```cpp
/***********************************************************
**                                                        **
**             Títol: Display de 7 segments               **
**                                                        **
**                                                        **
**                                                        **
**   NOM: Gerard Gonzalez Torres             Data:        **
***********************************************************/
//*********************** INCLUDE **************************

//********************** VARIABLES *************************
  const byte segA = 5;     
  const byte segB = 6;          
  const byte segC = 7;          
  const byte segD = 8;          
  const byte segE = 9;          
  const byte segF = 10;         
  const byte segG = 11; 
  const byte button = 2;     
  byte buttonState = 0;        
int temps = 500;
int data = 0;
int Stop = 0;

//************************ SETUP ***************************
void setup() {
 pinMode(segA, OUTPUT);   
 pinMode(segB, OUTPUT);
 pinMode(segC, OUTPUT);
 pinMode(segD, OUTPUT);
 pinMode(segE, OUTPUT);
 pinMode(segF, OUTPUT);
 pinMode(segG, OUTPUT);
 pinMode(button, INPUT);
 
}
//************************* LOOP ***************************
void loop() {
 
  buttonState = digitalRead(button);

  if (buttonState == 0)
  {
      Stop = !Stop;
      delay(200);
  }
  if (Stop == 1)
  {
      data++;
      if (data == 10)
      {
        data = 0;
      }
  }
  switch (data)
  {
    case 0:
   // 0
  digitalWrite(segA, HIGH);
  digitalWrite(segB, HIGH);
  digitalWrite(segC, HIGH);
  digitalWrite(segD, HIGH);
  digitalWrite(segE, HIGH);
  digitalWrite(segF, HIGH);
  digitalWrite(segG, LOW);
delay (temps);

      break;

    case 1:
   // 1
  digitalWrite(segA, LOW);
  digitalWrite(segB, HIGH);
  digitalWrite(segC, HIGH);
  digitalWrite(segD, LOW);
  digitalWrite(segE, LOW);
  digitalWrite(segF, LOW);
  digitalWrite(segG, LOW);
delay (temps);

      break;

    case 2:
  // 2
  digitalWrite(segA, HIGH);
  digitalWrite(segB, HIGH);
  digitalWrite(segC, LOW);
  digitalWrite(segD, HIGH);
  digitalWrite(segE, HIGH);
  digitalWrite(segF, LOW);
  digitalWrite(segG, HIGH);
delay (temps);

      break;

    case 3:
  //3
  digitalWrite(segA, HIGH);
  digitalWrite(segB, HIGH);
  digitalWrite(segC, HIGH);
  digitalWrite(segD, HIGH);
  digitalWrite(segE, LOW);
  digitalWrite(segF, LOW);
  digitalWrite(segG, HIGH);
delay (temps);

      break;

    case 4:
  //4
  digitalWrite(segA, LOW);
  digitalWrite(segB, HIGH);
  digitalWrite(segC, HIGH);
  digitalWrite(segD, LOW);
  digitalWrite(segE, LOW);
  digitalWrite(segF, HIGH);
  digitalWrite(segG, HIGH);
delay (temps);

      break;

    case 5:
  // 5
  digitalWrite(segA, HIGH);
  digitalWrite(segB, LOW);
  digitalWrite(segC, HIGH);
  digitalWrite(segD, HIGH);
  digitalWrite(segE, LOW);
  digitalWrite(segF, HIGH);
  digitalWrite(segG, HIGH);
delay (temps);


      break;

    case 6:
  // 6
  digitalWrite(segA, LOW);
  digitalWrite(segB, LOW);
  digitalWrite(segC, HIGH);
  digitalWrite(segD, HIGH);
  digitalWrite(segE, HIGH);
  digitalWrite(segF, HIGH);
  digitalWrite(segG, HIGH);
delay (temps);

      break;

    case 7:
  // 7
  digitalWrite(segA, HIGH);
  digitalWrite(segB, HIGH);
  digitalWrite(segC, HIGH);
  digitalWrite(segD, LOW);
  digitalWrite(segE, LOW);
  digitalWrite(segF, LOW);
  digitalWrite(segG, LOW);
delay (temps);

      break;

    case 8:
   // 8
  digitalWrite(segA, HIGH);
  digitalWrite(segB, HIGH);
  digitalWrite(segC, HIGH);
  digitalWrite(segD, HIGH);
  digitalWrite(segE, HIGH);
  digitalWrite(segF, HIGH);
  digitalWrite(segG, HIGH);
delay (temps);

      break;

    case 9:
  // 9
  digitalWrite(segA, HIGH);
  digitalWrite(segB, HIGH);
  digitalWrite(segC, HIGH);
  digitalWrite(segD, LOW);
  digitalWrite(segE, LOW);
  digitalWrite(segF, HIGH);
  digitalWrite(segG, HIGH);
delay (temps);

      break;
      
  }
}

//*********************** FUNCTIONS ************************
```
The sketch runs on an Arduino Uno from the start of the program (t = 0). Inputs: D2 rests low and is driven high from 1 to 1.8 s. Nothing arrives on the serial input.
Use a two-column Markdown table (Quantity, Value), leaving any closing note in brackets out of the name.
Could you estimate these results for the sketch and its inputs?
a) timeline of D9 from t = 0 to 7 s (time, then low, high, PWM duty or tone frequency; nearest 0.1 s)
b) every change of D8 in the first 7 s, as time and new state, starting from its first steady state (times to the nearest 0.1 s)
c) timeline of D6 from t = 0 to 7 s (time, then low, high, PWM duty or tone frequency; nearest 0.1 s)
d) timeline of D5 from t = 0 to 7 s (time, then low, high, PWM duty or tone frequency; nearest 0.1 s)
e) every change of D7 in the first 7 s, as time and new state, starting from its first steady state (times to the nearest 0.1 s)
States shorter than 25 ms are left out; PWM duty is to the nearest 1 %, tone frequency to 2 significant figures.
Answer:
| Quantity | Value |
|---|---|
| timeline of D9 from t = 0 to 7 s | 0 s low; 2.1 s high; 3.5 s low |
| every change of D8 in the first 7 s, as time and new state, starting from its first steady state | 0 s low; 2.1 s high; 4.9 s low; 6.3 s high |
| timeline of D6 from t = 0 to 7 s | 0 s low; 0.2 s high; 6.3 s low |
| timeline of D5 from t = 0 to 7 s | 0 s low; 2.1 s high; 4.9 s low; 6.3 s high |
| every change of D7 in the first 7 s, as time and new state, starting from its first steady state | 0 s low; 0.2 s high; 2.1 s low; 3.5 s high |
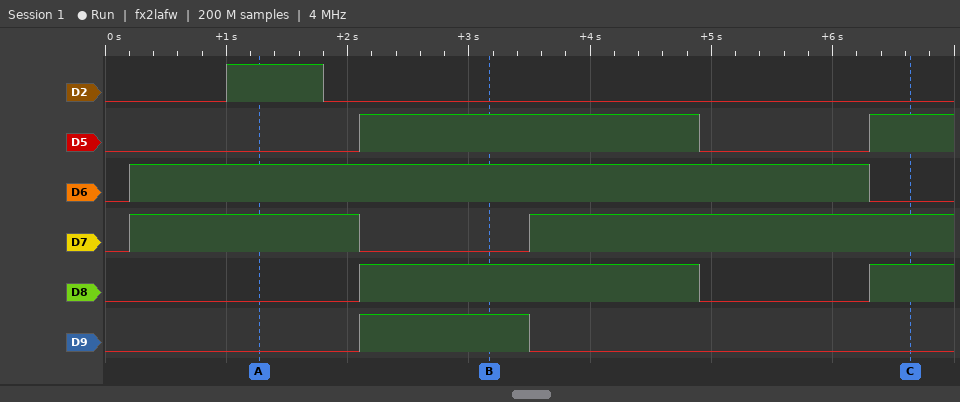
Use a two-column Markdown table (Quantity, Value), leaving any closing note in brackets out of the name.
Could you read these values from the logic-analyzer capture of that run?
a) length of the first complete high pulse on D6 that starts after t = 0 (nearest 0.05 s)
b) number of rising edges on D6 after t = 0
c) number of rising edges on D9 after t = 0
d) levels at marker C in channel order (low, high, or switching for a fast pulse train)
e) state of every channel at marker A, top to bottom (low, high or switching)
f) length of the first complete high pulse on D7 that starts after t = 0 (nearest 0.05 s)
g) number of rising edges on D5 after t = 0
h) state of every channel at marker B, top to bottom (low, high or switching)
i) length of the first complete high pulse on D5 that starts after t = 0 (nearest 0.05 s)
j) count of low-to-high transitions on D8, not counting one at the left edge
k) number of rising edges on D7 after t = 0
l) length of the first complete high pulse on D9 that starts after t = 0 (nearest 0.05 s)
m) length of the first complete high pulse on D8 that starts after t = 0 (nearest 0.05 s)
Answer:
| Quantity | Value |
|---|---|
| length of the first complete high pulse on D6 that starts after t = 0 | 6.10 s |
| number of rising edges on D6 after t = 0 | 1 |
| number of rising edges on D9 after t = 0 | 1 |
| levels at marker C in channel order | D2 low, D5 high, D6 low, D7 high, D8 high, D9 low |
| state of every channel at marker A, top to bottom | D2 high, D5 low, D6 high, D7 high, D8 low, D9 low |
| length of the first complete high pulse on D7 that starts after t = 0 | 1.90 s |
| number of rising edges on D5 after t = 0 | 2 |
| state of every channel at marker B, top to bottom | D2 low, D5 high, D6 high, D7 low, D8 high, D9 high |
| length of the first complete high pulse on D5 that starts after t = 0 | 2.80 s |
| count of low-to-high transitions on D8, not counting one at the left edge | 2 |
| number of rising edges on D7 after t = 0 | 2 |
| length of the first complete high pulse on D9 that starts after t = 0 | 1.40 s |
| length of the first complete high pulse on D8 that starts after t = 0 | 2.80 s |
